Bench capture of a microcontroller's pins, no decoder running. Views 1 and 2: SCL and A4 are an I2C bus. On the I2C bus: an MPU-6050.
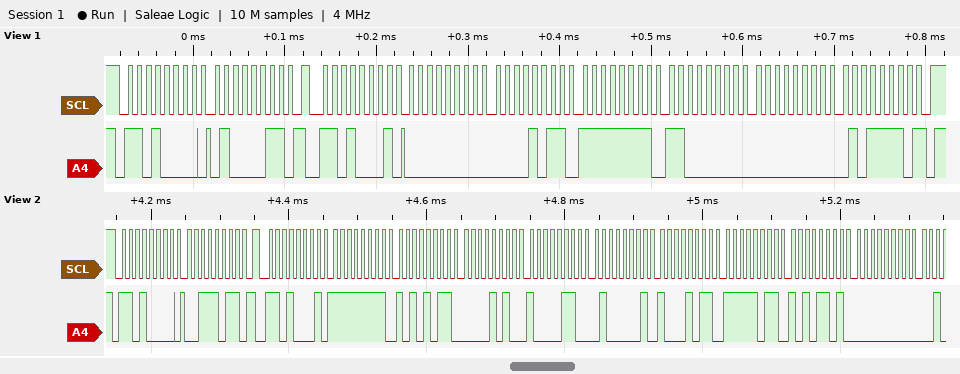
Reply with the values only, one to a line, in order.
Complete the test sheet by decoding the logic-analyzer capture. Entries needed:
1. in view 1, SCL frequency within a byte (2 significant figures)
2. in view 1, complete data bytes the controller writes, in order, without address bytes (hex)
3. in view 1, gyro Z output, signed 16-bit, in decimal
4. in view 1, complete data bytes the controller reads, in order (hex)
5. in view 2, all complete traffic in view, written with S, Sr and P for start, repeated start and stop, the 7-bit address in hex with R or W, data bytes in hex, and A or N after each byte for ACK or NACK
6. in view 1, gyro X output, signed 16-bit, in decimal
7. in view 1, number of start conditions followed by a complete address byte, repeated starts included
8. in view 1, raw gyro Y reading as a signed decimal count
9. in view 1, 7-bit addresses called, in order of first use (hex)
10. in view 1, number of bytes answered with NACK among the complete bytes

100 kHz
43
94
00 0B FF C0 00 5E
S 68W A 3B A Sr 68R A FF A AB A 0A A 86 A 41 A 8B A FB A AD A 00 A
11
2
-64
0x68
1
